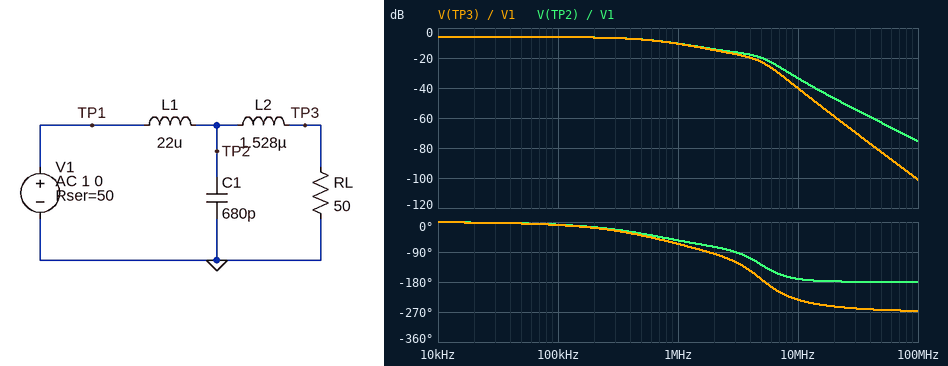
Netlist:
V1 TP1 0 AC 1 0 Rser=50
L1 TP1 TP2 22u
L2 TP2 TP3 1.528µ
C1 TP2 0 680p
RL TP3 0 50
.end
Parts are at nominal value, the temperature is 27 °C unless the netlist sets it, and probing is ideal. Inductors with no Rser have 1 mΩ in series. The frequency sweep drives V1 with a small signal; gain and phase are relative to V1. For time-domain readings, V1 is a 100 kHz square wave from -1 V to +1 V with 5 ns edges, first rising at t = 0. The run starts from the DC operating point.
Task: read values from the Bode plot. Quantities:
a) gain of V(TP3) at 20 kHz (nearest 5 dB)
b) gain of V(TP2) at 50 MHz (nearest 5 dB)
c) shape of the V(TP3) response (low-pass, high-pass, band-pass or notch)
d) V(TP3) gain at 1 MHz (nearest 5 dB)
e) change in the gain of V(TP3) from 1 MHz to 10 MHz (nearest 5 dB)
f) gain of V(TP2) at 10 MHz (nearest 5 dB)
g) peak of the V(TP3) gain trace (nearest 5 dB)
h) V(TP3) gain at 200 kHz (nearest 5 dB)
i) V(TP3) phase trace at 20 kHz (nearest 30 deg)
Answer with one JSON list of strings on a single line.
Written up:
["-5 dB", "-65 dB", "low-pass", "-10 dB", "-30 dB", "-35 dB", "-5 dB", "-5 dB", "0 deg"]
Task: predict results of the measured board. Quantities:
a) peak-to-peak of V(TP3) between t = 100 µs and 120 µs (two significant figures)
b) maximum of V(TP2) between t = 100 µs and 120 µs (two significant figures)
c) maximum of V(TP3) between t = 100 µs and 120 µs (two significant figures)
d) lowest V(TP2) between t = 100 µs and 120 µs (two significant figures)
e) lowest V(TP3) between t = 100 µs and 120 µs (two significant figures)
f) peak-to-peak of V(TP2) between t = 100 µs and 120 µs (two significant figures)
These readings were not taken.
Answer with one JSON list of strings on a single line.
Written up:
["1.0 V", "500 mV", "500 mV", "-500 mV", "-500 mV", "1.0 V"]
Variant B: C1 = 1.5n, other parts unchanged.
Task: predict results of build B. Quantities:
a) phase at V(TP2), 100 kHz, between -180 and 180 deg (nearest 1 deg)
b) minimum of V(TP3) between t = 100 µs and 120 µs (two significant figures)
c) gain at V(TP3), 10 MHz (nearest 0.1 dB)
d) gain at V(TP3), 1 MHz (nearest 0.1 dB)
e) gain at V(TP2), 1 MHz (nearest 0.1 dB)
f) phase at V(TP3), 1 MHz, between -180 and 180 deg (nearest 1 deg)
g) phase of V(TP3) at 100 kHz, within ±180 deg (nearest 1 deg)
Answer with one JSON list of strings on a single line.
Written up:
["-9 deg", "-500 mV", "-48.2 dB", "-10.2 dB", "-10.0 dB", "-79 deg", "-10 deg"]
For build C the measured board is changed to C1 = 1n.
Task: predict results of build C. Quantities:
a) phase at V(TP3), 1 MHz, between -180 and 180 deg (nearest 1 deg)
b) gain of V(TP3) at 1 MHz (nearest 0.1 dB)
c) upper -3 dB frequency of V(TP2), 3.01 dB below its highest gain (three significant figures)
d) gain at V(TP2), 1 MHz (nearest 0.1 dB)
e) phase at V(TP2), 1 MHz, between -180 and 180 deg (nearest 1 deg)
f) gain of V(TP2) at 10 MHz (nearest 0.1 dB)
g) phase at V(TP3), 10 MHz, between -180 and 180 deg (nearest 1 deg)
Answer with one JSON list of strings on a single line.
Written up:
["-71 deg", "-10.3 dB", "781 kHz", "-10.2 dB", "-60 deg", "-37.5 dB", "124 deg"]
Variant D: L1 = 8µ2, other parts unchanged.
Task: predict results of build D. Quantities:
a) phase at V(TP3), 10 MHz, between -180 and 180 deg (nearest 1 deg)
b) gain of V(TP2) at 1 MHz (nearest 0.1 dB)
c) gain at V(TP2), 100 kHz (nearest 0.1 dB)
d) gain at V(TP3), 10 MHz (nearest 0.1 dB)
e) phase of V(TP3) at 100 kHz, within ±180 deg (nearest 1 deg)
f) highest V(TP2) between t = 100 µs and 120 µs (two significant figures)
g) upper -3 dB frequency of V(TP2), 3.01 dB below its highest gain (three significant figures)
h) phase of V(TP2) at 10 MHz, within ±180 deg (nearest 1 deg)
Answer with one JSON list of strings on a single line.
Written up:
["131 deg", "-6.8 dB", "-6.0 dB", "-31.3 dB", "-4 deg", "500 mV", "3.40 MHz", "-167 deg"]
